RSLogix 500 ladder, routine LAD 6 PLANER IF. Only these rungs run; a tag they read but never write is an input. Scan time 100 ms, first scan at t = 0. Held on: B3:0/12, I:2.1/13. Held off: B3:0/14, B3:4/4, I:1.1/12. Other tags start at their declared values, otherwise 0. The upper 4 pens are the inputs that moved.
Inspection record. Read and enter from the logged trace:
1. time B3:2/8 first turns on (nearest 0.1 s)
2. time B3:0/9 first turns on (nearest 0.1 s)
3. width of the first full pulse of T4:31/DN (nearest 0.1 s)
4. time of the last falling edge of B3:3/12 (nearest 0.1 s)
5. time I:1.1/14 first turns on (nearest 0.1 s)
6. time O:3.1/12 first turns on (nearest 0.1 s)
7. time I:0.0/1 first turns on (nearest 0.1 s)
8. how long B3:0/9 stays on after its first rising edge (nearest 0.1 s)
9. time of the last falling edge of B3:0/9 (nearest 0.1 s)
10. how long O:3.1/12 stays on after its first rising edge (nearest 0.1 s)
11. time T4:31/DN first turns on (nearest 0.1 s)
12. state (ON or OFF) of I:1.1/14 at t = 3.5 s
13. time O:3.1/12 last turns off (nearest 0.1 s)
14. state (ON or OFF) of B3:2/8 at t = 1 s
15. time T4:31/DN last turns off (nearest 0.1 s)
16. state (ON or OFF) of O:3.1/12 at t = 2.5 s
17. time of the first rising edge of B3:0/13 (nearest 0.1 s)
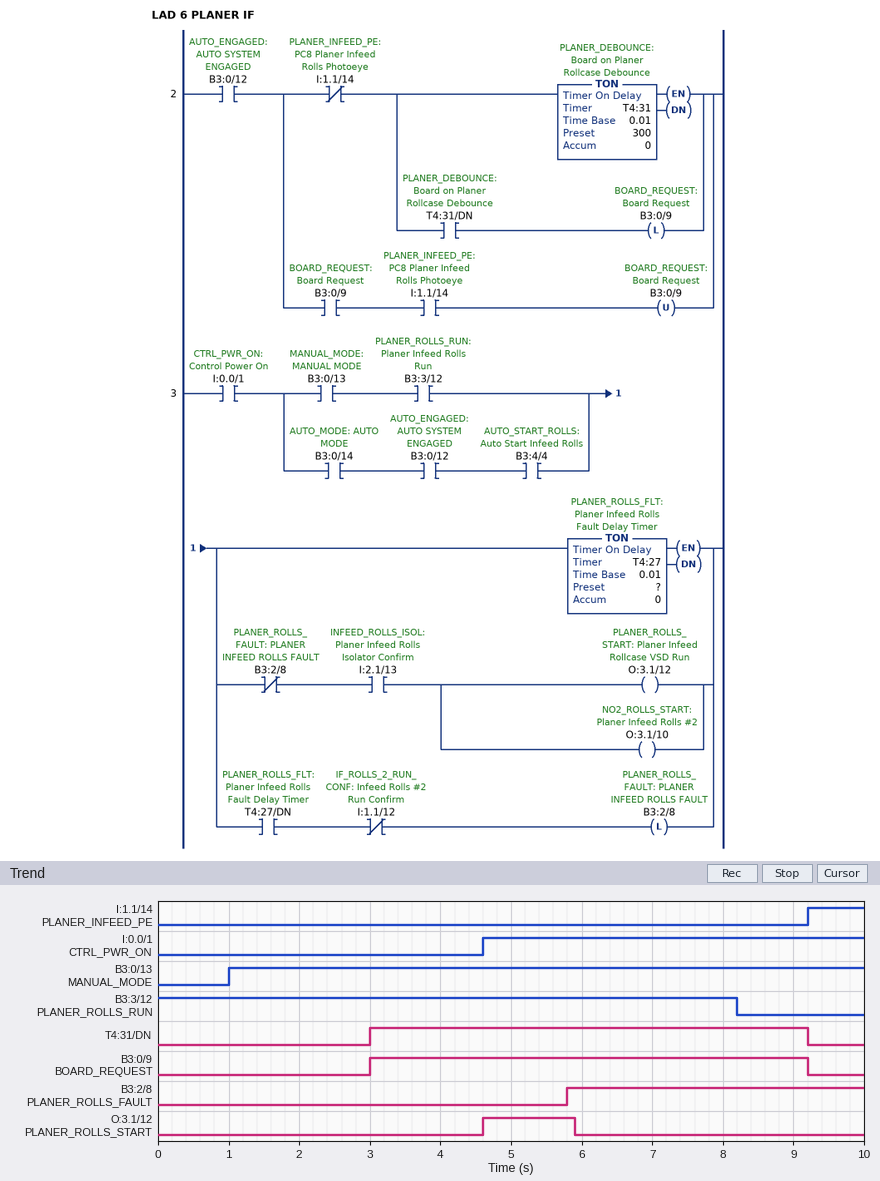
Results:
5.8 s
3.0 s
6.2 s
8.2 s
9.2 s
4.6 s
4.6 s
6.2 s
9.2 s
1.3 s
3.0 s
OFF
5.9 s
OFF
9.2 s
OFF
1.0 s
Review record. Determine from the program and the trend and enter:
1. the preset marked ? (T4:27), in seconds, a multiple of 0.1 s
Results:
1.2 s
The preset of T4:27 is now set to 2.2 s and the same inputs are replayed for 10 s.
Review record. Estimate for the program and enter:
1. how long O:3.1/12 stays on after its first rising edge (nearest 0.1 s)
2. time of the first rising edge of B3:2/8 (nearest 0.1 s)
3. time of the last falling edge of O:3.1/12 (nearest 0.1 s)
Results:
2.3 s
6.8 s
6.9 s
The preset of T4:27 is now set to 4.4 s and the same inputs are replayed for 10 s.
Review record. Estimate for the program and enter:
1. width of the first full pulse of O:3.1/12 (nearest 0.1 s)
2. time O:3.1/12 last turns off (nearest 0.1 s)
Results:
3.6 s
8.2 s
